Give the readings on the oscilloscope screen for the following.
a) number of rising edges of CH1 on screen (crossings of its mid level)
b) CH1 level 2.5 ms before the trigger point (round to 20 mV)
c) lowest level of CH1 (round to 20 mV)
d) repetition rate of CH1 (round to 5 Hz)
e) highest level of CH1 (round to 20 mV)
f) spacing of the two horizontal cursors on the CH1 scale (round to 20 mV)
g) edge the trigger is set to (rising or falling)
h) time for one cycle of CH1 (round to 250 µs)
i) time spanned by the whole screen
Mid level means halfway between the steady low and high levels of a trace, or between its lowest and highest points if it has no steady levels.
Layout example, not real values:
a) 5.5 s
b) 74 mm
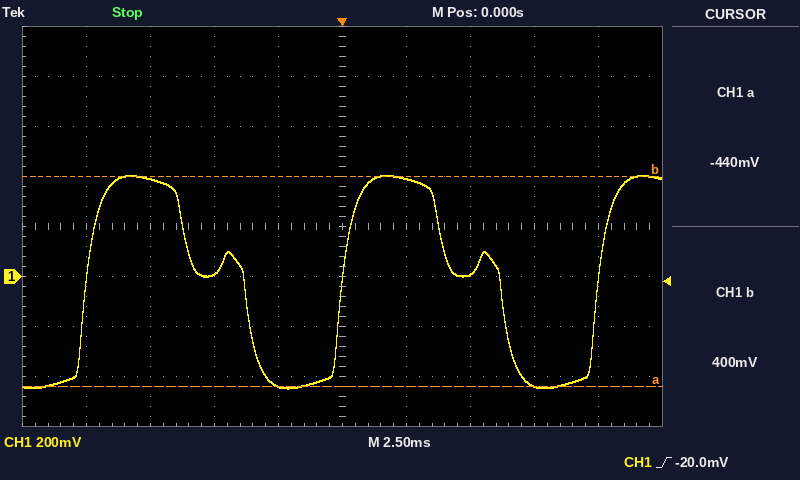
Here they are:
a) 3
b) -440 mV
c) -440 mV
d) 100 Hz
e) 400 mV
f) 840 mV
g) rising
h) 10.00 ms
i) 25 ms
